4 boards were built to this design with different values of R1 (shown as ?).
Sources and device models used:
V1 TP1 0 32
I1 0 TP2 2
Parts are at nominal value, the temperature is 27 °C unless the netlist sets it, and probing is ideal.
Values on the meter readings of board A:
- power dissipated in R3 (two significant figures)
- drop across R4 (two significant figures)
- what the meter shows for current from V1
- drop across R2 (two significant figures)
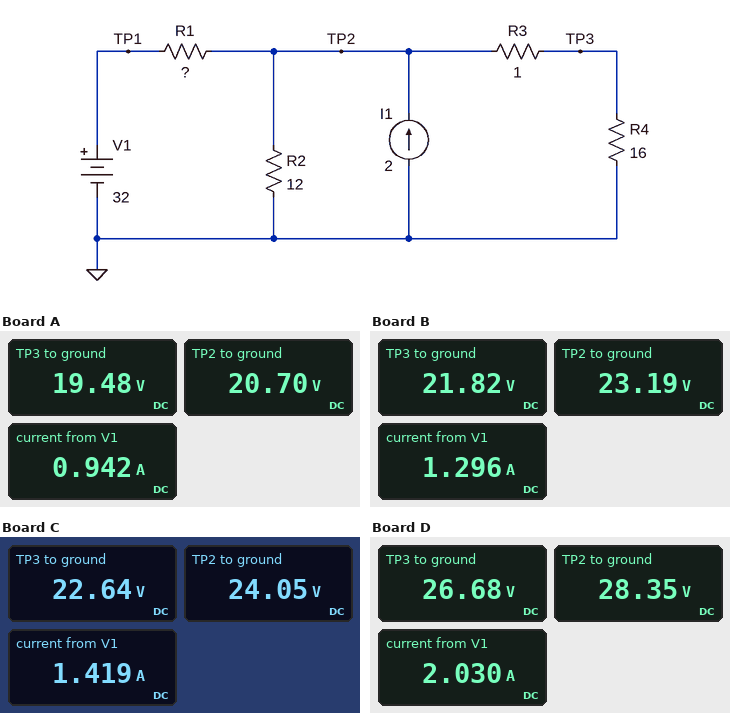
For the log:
1.5 W
19 V
0.942 A
21 V
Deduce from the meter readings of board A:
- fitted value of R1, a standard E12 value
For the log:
12 Ω
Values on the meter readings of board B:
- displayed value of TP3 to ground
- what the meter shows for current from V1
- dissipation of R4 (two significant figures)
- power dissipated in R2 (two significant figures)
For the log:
21.82 V
1.296 A
30 W
45 W
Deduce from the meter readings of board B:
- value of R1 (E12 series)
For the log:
6.8 Ω
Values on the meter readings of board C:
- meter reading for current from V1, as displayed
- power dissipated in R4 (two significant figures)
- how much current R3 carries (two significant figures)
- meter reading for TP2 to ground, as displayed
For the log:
1.419 A
32 W
1.4 A
24.05 V
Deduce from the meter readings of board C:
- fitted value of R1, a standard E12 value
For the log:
5.6 Ω
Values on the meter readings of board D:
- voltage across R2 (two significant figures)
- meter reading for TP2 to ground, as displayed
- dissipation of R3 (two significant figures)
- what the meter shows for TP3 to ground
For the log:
28 V
28.35 V
2.8 W
26.68 V
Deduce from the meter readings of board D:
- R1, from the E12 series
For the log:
1.8 Ω
